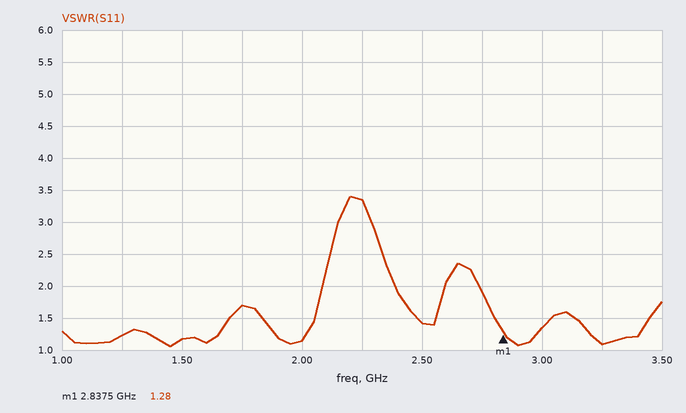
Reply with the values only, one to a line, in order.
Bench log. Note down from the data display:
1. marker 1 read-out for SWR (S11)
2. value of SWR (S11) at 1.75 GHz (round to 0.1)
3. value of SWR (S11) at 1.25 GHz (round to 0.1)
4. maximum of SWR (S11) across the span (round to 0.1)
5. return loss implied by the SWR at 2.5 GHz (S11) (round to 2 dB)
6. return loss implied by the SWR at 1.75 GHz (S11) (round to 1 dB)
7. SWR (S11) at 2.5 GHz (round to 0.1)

1.28
1.7
1.2
3.4
16 dB
12 dB
1.4
